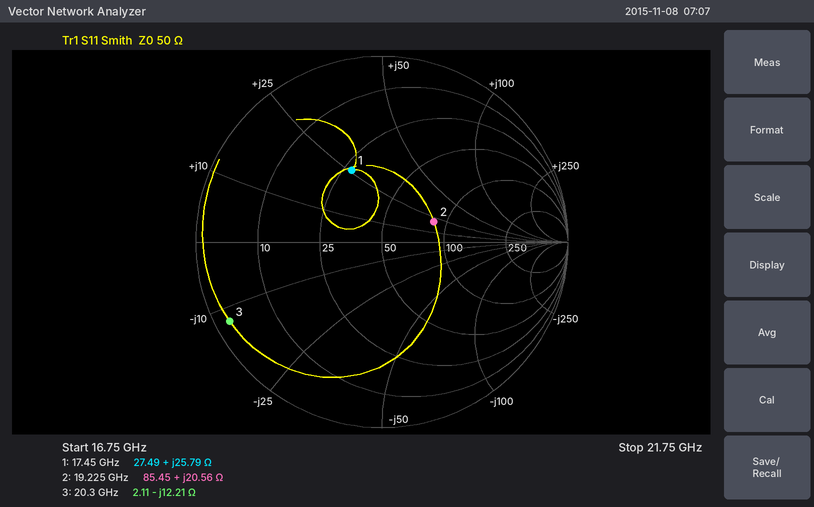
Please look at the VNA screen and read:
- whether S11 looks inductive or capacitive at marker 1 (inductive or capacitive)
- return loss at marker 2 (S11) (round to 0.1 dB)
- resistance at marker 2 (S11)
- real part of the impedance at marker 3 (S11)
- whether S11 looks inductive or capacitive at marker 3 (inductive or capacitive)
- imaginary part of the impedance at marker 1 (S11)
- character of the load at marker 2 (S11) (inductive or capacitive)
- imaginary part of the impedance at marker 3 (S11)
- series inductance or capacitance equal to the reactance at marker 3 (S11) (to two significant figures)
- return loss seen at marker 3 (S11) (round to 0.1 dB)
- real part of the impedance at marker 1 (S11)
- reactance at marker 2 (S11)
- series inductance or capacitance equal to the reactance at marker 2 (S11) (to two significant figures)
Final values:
inductive
10.5 dB
85.45 Ω
2.11 Ω
capacitive
+25.79 Ω
inductive
-12.21 Ω
640 fF
0.7 dB
27.49 Ω
+20.56 Ω
170 pH
